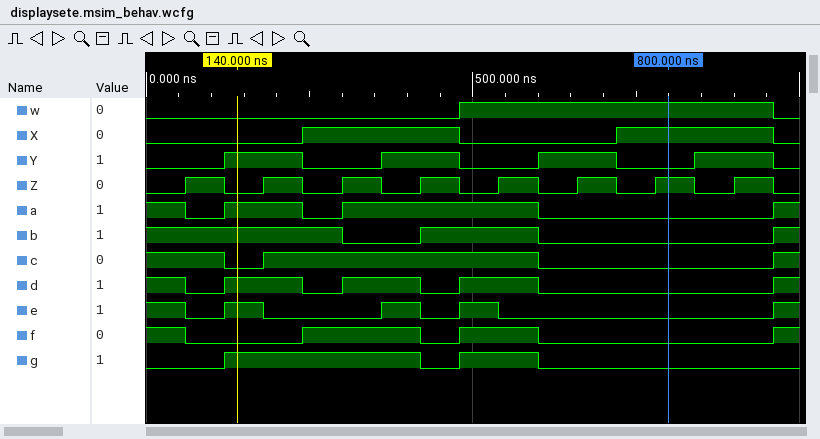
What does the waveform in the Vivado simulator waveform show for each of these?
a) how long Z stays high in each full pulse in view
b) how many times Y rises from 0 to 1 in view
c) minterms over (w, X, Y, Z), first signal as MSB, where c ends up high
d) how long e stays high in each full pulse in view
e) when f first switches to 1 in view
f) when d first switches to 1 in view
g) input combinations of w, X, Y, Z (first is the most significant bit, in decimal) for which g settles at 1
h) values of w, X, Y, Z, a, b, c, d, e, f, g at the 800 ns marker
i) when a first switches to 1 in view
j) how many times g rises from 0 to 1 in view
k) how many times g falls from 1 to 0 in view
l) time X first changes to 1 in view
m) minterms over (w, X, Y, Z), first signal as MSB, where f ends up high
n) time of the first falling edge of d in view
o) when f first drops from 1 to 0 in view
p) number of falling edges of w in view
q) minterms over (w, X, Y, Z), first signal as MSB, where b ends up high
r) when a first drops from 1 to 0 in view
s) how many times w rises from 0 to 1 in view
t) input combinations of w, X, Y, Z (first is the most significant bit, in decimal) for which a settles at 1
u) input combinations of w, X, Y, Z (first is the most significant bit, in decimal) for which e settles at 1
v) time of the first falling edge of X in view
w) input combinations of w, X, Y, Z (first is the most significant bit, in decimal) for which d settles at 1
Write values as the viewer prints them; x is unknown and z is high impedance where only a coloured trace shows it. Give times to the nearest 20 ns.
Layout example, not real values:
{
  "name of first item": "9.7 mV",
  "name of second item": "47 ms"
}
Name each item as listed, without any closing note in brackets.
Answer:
{
  "how long Z stays high in each full pulse in view": "60 ns, 60 ns, 60 ns, 60 ns, 60 ns, 60 ns, 60 ns, 60 ns",
  "how many times Y rises from 0 to 1 in view": "4",
  "minterms over (w, X, Y, Z), first signal as MSB, where c ends up high": "0, 1, 3, 4, 5, 6, 7, 8, 9",
  "how long e stays high in each full pulse in view": "60 ns, 60 ns, 60 ns",
  "when f first switches to 1 in view": "240 ns",
  "when d first switches to 1 in view": "120 ns",
  "input combinations of w, X, Y, Z (first is the most significant bit, in decimal) for which g settles at 1": "2, 3, 4, 5, 6, 8, 9",
  "values of w, X, Y, Z, a, b, c, d, e, f, g at the 800 ns marker": "w=1, X=1, Y=0, Z=1, a=0, b=0, c=0, d=0, e=0, f=0, g=0",
  "when a first switches to 1 in view": "120 ns",
  "how many times g rises from 0 to 1 in view": "2",
  "how many times g falls from 1 to 0 in view": "2",
  "time X first changes to 1 in view": "240 ns",
  "minterms over (w, X, Y, Z), first signal as MSB, where f ends up high": "0, 4, 5, 6, 8, 9",
  "time of the first falling edge of d in view": "60 ns",
  "when f first drops from 1 to 0 in view": "60 ns",
  "number of falling edges of w in view": "1",
  "minterms over (w, X, Y, Z), first signal as MSB, where b ends up high": "0, 1, 2, 3, 4, 7, 8, 9",
  "when a first drops from 1 to 0 in view": "60 ns",
  "how many times w rises from 0 to 1 in view": "1",
  "input combinations of w, X, Y, Z (first is the most significant bit, in decimal) for which a settles at 1": "0, 2, 3, 5, 6, 7, 8, 9",
  "input combinations of w, X, Y, Z (first is the most significant bit, in decimal) for which e settles at 1": "0, 2, 6, 8",
  "time of the first falling edge of X in view": "480 ns",
  "input combinations of w, X, Y, Z (first is the most significant bit, in decimal) for which d settles at 1": "0, 2, 3, 5, 6, 8, 9"
}
